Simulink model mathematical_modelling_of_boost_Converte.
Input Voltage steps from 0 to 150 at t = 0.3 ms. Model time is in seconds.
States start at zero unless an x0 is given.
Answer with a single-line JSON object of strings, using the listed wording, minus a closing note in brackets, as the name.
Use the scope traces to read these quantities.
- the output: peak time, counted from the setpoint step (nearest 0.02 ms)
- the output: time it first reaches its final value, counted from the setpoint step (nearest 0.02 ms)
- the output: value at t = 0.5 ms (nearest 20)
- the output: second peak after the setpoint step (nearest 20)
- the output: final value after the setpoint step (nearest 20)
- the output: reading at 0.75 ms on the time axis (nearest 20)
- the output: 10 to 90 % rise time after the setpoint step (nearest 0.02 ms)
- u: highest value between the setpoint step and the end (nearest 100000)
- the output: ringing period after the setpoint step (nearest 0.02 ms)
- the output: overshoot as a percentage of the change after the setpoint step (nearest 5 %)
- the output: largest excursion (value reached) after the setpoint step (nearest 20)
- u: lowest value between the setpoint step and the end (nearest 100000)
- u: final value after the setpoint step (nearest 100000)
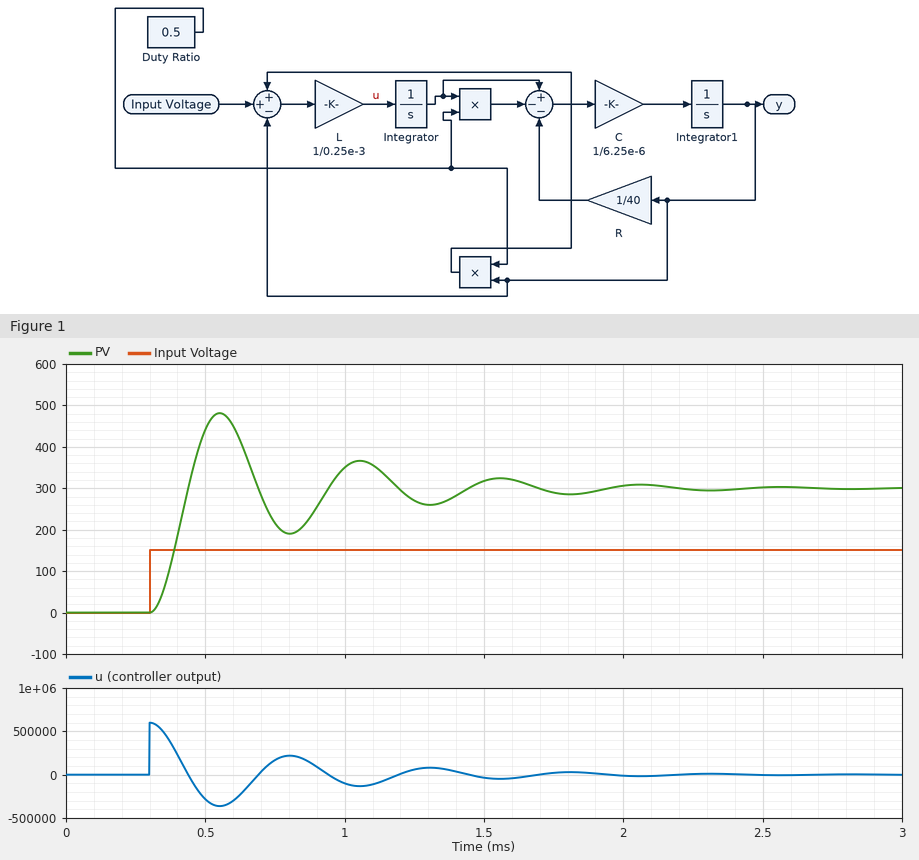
{"the output: peak time, counted from the setpoint step": "0.26 ms", "the output: time it first reaches its final value, counted from the setpoint step": "0.14 ms", "the output: value at t = 0.5 ms": "440", "the output: second peak after the setpoint step": "360", "the output: final value after the setpoint step": "300", "the output: reading at 0.75 ms on the time axis": "220", "the output: 10 to 90 % rise time after the setpoint step": "0.10 ms", "u: highest value between the setpoint step and the end": "600000", "the output: ringing period after the setpoint step": "0.50 ms", "the output: overshoot as a percentage of the change after the setpoint step": "60 %", "the output: largest excursion (value reached) after the setpoint step": "480", "u: lowest value between the setpoint step and the end": "-400000", "u: final value after the setpoint step": "0"}
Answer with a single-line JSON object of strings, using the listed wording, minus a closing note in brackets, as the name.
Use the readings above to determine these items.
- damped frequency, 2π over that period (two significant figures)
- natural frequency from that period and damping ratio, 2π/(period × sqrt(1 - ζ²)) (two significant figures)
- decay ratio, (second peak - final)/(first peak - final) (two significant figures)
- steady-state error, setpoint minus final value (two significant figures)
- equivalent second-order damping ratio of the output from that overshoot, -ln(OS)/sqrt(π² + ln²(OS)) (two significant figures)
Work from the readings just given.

{"damped frequency, 2π over that period": "13 rad/ms", "natural frequency from that period and damping ratio, 2π/(period × sqrt(1 - ζ²))": "13 rad/ms", "decay ratio, (second peak - final)/(first peak - final)": "0.33", "steady-state error, setpoint minus final value": "-150", "equivalent second-order damping ratio of the output from that overshoot, -ln(OS)/sqrt(π² + ln²(OS))": "0.16"}
